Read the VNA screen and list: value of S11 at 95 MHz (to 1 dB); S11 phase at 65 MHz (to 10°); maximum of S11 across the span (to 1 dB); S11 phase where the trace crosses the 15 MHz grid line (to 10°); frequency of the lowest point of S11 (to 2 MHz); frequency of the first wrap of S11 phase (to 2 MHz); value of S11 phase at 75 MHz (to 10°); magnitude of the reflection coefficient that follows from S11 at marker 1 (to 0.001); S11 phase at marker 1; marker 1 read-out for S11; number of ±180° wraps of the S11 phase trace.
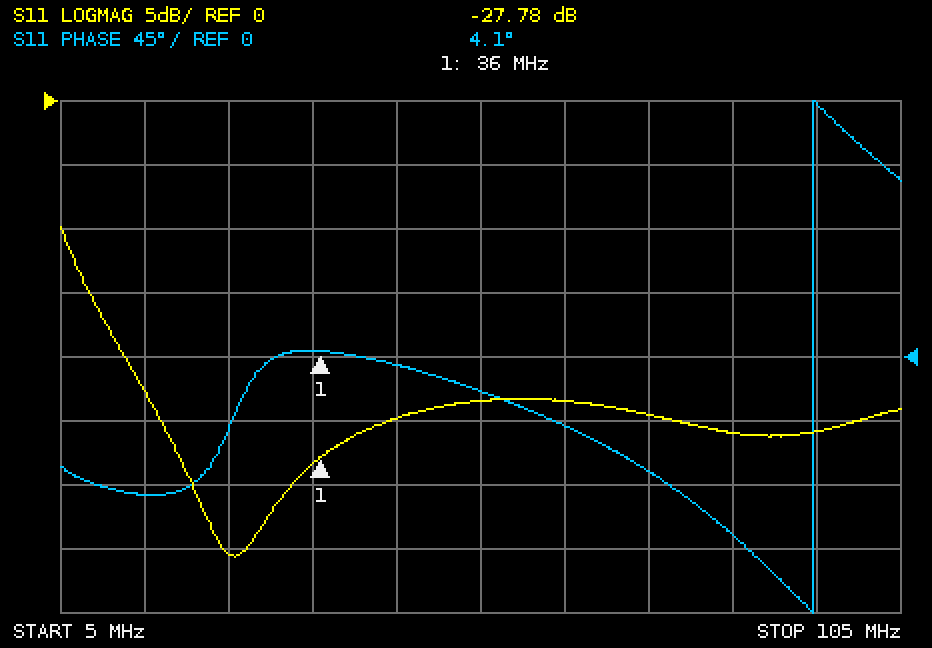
-26 dB
-50°
-10 dB
-100°
26 MHz
94 MHz
-80°
0.041
4.1°
-27.78 dB
1
